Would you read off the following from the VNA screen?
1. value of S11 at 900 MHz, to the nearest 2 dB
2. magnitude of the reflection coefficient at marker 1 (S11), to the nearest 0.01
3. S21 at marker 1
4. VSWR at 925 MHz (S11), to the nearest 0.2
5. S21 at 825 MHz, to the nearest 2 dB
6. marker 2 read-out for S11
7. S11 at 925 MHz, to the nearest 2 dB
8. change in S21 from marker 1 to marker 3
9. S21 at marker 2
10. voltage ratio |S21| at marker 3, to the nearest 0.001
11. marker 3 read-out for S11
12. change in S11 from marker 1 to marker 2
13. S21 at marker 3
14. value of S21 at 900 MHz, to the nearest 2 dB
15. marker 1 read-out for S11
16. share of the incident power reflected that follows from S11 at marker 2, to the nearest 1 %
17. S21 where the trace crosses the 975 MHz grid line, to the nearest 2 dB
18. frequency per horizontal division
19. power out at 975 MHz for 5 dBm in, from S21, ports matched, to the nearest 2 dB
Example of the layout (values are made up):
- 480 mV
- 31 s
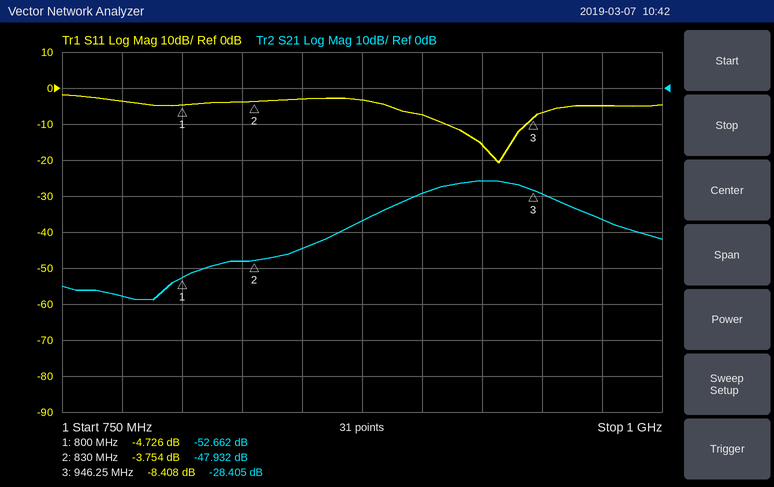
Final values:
- -8 dB
- 0.58
- -52.662 dB
- 1.4
- -48 dB
- -3.754 dB
- -16 dB
- 24.257 dB
- -47.932 dB
- 0.038
- -8.408 dB
- 0.972 dB
- -28.405 dB
- -30 dB
- -4.726 dB
- 42 %
- -36 dB
- 25 MHz
- -32 dBm
